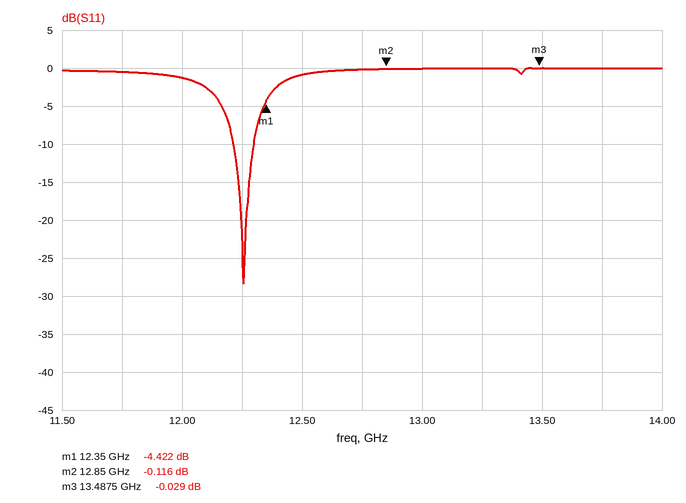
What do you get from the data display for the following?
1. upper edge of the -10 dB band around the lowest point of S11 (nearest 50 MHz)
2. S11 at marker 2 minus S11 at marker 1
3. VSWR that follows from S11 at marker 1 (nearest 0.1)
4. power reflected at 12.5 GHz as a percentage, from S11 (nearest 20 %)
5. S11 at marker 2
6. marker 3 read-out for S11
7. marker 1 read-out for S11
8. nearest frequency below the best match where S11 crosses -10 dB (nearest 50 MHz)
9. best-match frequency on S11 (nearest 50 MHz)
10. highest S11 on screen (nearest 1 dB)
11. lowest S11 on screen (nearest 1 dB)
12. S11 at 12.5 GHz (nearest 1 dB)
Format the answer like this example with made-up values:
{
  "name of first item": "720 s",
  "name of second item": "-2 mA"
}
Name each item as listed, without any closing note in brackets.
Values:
{
  "upper edge of the -10 dB band around the lowest point of S11": "12.30 GHz",
  "S11 at marker 2 minus S11 at marker 1": "4.306 dB",
  "VSWR that follows from S11 at marker 1": "4.0",
  "power reflected at 12.5 GHz as a percentage, from S11": "80 %",
  "S11 at marker 2": "-0.116 dB",
  "marker 3 read-out for S11": "-0.029 dB",
  "marker 1 read-out for S11": "-4.422 dB",
  "nearest frequency below the best match where S11 crosses -10 dB": "12.20 GHz",
  "best-match frequency on S11": "12.25 GHz",
  "highest S11 on screen": "0 dB",
  "lowest S11 on screen": "-28 dB",
  "S11 at 12.5 GHz": "-1 dB"
}
